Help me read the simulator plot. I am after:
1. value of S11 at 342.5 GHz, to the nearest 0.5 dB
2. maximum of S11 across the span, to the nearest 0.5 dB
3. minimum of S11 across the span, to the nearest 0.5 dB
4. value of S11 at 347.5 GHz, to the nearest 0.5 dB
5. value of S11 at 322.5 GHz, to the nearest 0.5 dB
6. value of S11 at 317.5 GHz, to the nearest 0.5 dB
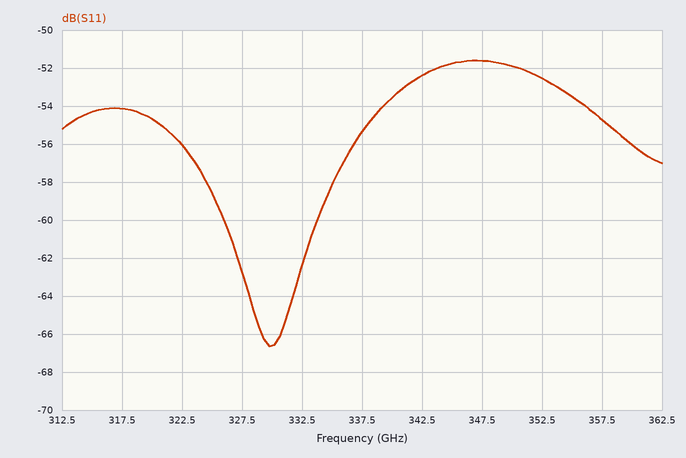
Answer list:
-52.5 dB
-51.5 dB
-66.5 dB
-51.5 dB
-56.0 dB
-54.0 dB
